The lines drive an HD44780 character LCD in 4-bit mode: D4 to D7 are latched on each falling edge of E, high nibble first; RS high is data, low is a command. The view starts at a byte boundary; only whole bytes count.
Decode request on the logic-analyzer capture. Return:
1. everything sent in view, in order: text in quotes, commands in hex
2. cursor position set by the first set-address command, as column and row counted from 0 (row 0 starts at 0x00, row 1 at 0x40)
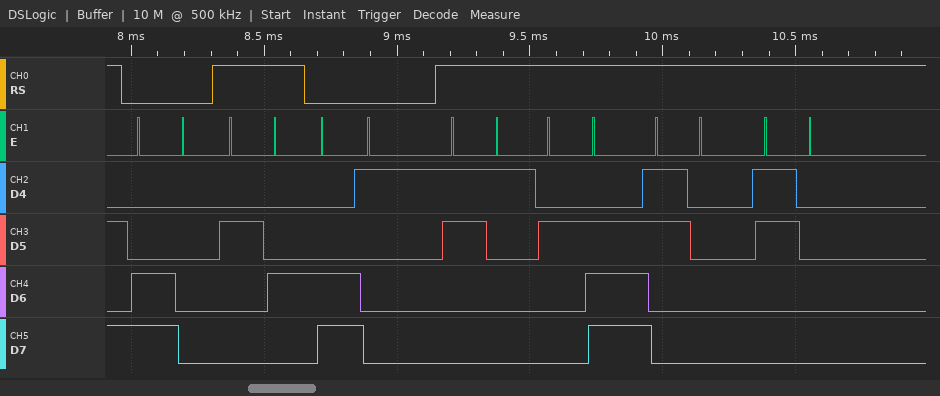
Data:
0xC0 "$" 0xC1 "1.00"
column 0, row 1
